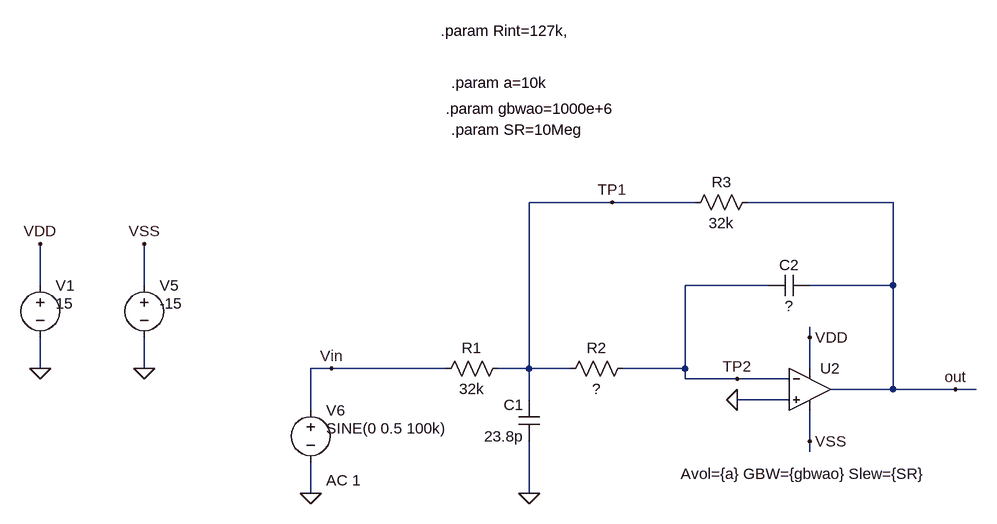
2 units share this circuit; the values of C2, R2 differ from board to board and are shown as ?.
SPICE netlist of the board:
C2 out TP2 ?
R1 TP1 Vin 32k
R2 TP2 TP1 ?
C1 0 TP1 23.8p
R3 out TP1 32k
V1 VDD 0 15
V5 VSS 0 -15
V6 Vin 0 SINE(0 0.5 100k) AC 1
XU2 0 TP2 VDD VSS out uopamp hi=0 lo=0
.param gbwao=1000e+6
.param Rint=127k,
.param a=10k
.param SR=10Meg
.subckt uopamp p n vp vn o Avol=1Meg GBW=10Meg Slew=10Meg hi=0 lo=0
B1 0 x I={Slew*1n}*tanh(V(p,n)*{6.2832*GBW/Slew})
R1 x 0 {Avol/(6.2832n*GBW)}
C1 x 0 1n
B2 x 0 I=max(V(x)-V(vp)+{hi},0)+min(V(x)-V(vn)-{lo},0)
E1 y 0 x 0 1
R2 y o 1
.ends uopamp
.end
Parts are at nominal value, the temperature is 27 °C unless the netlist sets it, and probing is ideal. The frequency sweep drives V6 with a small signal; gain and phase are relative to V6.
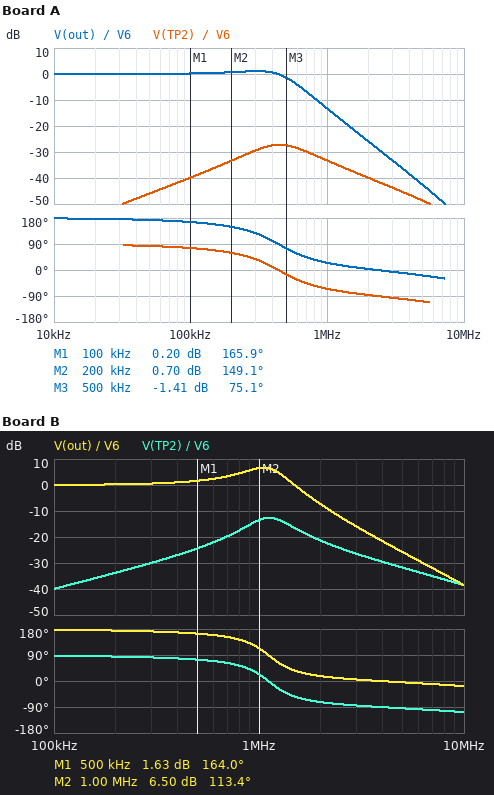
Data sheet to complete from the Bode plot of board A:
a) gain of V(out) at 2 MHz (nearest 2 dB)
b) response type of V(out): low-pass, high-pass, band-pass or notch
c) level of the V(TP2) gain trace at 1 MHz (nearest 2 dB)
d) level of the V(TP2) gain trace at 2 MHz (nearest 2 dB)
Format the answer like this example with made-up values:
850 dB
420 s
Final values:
-26 dB
low-pass
-34 dB
-40 dB
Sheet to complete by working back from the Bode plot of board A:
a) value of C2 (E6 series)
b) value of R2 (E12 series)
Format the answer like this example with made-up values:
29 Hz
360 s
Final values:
1.5 pF
100 kΩ
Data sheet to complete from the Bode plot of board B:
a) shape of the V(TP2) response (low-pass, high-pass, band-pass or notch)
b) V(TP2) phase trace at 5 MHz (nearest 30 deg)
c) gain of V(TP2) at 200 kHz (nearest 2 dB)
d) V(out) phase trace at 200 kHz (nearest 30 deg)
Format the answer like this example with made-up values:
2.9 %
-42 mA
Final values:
band-pass
-90 deg
-34 dB
180 deg
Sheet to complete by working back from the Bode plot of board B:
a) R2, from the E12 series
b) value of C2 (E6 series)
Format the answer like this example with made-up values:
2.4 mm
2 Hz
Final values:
15 kΩ
680 fF
